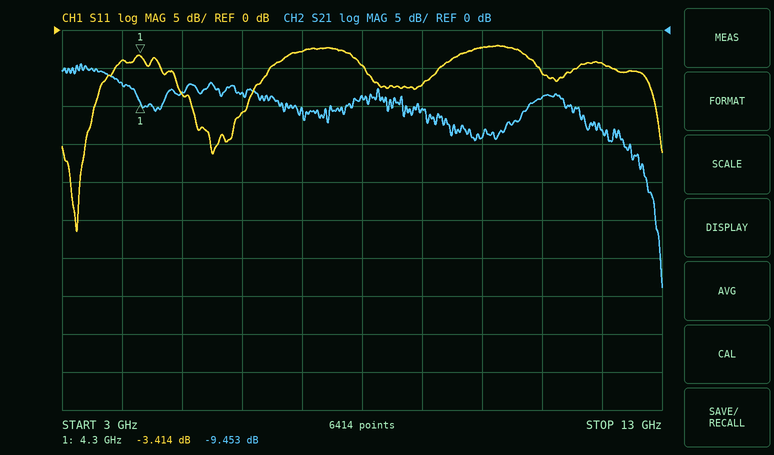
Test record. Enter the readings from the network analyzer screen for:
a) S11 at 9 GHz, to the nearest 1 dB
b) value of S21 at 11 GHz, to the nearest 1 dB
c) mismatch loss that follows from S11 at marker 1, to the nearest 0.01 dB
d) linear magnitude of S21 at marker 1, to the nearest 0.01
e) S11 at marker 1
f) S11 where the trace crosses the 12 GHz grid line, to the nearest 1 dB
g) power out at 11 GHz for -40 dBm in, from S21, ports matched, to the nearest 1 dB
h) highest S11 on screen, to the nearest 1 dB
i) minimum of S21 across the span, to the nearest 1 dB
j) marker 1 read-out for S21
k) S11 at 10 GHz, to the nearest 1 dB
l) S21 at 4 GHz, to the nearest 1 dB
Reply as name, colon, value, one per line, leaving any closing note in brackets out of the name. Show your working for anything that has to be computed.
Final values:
S11 at 9 GHz, to the nearest 1 dB: -7 dB
value of S21 at 11 GHz, to the nearest 1 dB: -9 dB
mismatch loss that follows from S11 at marker 1, to the nearest 0.01 dB: −10 log10(1 − 10^(-3.414/10)) ≈ 2.64 dB
linear magnitude of S21 at marker 1, to the nearest 0.01: 10^(-9.453/20) ≈ 0.34
S11 at marker 1: -3.414 dB
S11 where the trace crosses the 12 GHz grid line, to the nearest 1 dB: -4 dB
power out at 11 GHz for -40 dBm in, from S21, ports matched, to the nearest 1 dB: -40 dBm + (-9 dB) = -49 dBm
highest S11 on screen, to the nearest 1 dB: -2 dB
minimum of S21 across the span, to the nearest 1 dB: -34 dB
marker 1 read-out for S21: -9.453 dB
S11 at 10 GHz, to the nearest 1 dB: -2 dB
S21 at 4 GHz, to the nearest 1 dB: -7 dB
